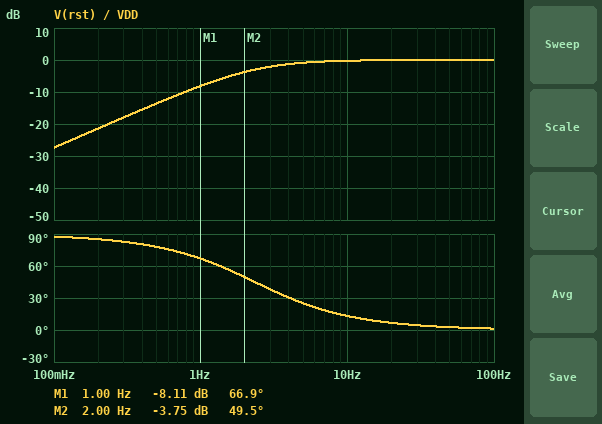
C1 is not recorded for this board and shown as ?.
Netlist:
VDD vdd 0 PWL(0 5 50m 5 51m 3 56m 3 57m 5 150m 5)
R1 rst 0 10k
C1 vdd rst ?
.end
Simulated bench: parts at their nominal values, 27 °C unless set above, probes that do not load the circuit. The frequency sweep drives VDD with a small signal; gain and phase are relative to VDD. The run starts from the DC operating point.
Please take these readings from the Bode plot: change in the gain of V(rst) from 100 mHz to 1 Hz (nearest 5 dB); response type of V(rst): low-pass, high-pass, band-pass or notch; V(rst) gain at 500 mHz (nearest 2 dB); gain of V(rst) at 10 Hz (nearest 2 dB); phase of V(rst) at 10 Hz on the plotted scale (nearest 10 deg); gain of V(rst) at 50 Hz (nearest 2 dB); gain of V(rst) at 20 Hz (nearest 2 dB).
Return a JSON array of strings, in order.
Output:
["20 dB", "high-pass", "-14 dB", "0 dB", "10 deg", "0 dB", "0 dB"]
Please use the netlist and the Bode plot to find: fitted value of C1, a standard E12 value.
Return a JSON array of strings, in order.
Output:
["6.8 µF"]
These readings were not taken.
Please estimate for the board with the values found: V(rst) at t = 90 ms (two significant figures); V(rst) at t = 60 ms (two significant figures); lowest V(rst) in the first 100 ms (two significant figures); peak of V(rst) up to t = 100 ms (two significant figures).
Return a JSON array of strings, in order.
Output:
["100 mV", "160 mV", "-2.0 V", "170 mV"]
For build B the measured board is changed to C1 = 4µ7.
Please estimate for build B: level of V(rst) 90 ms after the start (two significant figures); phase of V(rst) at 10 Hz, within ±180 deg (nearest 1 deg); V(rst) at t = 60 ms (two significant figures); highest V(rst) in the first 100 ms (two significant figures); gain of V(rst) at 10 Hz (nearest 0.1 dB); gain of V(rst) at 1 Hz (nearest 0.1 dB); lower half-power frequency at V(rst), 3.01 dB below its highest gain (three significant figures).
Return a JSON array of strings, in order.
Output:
["120 mV", "19 deg", "220 mV", "240 mV", "-0.5 dB", "-11.0 dB", "3.39 Hz"]
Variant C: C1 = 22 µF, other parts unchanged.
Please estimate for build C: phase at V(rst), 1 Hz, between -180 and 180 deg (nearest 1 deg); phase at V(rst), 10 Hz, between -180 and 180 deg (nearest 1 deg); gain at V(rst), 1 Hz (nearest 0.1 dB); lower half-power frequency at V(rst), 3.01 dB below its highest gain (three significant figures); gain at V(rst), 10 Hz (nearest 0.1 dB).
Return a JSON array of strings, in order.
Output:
["36 deg", "4 deg", "-1.8 dB", "723 mHz", "0 dB"]
